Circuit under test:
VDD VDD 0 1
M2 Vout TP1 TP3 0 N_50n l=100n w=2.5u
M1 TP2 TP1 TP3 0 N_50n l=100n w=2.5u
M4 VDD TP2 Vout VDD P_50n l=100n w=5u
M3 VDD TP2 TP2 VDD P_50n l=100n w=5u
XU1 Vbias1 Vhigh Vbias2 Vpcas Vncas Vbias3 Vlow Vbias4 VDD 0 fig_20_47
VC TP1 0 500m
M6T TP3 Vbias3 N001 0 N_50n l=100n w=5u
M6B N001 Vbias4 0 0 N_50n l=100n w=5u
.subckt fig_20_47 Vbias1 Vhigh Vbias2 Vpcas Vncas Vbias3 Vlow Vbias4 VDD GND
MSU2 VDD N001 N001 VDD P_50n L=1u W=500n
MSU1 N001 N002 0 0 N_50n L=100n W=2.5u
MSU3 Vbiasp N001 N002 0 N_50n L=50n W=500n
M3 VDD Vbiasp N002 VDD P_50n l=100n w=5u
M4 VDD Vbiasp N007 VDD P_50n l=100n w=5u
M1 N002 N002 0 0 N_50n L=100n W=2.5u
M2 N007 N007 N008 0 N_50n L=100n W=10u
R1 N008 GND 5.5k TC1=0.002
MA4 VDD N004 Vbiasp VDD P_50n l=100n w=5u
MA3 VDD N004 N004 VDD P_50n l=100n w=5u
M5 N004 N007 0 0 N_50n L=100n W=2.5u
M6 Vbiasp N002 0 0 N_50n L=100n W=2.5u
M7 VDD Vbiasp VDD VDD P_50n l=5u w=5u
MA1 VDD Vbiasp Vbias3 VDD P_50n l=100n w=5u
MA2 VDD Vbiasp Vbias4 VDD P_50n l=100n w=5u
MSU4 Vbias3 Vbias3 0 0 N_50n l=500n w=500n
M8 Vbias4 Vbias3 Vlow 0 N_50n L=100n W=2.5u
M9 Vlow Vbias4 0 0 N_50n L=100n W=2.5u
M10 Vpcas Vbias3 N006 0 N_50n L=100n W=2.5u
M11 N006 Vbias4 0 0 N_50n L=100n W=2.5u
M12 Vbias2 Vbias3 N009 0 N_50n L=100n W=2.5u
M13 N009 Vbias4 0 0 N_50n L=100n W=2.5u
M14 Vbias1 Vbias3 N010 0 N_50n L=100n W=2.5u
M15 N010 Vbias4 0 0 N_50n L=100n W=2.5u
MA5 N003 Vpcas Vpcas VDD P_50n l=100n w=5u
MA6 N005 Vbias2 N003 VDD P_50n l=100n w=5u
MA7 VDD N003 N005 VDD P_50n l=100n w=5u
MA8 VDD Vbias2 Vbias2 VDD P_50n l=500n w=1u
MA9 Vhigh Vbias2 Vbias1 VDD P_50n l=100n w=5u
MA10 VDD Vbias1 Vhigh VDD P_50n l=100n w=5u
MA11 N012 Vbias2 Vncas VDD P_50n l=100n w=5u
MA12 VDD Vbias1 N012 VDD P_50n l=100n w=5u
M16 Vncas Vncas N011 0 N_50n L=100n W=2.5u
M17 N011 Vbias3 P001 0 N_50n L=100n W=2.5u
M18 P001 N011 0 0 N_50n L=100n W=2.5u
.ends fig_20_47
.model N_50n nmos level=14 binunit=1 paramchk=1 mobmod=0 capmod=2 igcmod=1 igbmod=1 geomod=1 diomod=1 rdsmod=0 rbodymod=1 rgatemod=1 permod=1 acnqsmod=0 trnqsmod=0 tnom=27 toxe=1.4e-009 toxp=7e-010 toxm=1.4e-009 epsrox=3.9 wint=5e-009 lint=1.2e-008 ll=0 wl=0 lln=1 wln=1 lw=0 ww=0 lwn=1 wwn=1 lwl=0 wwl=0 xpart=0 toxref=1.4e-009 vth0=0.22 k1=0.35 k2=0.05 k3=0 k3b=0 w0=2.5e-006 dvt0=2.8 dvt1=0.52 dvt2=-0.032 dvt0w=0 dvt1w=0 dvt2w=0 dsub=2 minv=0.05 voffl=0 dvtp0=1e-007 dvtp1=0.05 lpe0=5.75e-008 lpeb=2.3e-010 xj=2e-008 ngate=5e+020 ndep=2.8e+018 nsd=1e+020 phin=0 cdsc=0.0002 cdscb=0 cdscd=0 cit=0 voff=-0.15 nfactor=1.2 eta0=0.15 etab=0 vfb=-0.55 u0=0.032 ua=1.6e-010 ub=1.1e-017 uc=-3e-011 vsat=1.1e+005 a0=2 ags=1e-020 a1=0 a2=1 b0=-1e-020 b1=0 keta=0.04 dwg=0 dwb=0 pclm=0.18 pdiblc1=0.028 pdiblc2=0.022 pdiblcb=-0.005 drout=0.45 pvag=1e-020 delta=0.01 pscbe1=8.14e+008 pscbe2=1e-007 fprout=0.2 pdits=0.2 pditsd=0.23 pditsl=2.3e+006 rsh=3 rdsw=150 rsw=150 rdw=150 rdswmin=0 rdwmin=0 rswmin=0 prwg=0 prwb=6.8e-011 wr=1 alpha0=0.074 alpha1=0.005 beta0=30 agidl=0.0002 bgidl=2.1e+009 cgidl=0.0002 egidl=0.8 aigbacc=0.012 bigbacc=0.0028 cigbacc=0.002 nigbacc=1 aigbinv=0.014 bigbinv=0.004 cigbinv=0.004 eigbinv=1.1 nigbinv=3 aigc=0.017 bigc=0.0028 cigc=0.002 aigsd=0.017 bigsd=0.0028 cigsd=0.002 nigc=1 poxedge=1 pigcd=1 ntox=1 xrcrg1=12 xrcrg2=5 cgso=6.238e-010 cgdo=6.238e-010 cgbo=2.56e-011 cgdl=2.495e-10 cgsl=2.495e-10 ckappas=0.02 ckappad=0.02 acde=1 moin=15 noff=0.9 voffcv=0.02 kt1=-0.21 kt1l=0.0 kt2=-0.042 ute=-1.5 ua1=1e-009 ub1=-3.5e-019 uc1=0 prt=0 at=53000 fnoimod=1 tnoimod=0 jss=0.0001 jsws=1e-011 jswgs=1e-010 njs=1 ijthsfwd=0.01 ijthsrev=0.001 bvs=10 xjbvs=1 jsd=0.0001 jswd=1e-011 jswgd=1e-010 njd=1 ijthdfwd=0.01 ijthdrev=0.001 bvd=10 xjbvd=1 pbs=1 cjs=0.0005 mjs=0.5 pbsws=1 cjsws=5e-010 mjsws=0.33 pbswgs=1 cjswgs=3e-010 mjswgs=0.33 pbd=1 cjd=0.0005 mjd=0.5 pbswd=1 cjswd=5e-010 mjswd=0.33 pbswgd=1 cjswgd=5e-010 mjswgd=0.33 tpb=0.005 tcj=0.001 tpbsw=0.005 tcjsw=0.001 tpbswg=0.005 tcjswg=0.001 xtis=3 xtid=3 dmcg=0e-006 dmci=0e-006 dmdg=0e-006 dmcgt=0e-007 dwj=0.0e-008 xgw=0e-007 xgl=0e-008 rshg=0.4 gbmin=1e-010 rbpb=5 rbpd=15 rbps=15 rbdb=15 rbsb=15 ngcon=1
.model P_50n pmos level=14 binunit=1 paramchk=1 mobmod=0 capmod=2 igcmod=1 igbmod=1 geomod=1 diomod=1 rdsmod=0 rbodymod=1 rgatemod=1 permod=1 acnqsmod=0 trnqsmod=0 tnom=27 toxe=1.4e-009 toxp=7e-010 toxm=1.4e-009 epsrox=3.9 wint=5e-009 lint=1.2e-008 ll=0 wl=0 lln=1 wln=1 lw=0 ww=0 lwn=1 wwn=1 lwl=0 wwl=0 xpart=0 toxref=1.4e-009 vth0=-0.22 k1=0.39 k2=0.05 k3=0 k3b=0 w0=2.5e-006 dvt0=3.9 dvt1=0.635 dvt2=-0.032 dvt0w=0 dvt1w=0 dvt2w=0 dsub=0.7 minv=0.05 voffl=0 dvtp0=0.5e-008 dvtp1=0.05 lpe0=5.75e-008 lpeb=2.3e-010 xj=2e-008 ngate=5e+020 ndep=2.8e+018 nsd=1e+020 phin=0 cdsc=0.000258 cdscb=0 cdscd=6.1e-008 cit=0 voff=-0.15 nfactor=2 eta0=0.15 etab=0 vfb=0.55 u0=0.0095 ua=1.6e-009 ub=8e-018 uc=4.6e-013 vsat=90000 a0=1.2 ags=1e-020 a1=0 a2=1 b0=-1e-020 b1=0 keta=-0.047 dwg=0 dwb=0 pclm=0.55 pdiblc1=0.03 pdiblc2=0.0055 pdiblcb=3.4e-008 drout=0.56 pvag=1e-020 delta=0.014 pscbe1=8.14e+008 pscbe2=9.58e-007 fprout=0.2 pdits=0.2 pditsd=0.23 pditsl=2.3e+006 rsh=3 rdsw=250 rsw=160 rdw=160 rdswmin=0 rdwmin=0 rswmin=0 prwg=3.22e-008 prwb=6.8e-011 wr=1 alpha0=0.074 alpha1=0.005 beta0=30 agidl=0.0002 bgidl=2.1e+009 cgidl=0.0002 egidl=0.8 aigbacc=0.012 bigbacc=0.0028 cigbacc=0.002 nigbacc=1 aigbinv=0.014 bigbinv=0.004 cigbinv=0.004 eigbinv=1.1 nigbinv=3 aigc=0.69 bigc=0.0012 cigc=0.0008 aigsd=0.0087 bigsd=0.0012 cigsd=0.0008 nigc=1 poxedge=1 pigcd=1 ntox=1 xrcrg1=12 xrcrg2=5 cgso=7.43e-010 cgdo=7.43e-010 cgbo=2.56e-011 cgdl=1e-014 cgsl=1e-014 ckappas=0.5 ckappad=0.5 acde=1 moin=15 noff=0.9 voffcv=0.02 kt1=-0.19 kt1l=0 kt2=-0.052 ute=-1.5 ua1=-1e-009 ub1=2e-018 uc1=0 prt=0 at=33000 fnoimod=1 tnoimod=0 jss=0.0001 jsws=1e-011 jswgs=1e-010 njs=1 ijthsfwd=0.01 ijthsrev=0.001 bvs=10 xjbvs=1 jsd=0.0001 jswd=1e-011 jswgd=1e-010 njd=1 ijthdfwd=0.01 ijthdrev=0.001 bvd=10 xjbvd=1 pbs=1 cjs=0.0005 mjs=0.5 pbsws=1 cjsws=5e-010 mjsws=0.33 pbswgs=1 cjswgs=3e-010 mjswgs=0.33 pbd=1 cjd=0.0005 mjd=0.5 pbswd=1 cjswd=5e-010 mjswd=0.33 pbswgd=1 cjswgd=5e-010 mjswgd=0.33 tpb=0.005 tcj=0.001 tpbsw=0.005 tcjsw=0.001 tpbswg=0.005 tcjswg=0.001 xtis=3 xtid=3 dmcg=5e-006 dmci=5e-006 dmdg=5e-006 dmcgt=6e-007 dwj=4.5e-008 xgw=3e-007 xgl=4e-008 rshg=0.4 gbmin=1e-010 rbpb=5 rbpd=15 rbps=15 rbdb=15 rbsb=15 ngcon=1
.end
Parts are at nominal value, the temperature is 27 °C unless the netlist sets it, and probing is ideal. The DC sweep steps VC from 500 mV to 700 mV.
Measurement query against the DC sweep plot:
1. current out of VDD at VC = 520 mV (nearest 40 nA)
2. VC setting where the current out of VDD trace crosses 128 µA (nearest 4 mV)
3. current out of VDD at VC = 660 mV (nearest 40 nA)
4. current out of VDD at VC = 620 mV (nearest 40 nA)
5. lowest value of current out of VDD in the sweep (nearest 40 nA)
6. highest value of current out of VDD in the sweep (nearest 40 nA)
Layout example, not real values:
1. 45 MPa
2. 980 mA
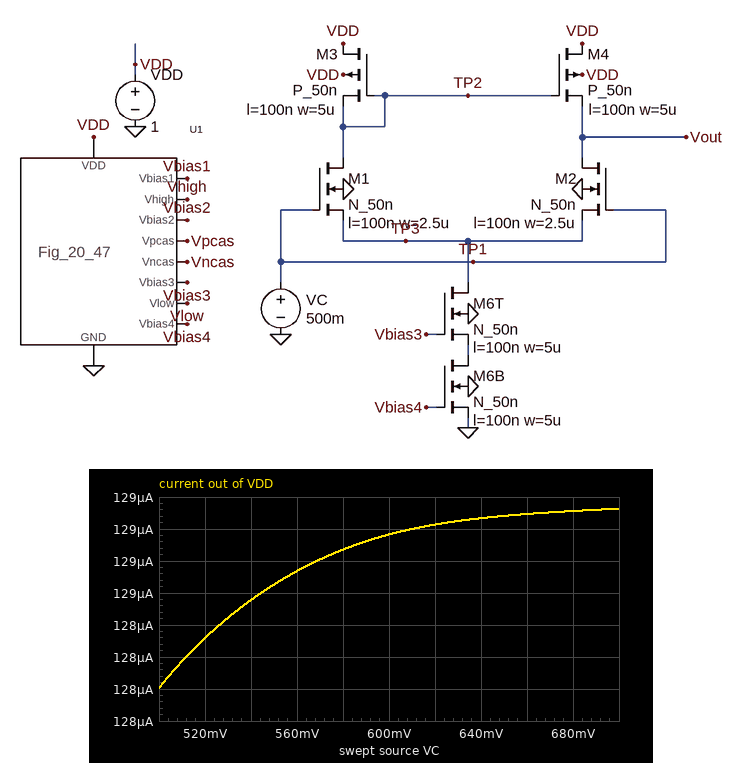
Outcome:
1. 128.32 µA
2. 512 mV
3. 129.08 µA
4. 129.04 µA
5. 128.00 µA
6. 129.12 µA
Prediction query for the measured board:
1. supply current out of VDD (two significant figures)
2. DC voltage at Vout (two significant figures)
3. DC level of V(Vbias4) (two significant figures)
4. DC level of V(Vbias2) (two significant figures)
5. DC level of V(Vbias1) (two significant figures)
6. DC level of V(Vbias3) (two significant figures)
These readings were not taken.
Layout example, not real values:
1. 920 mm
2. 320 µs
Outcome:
1. 130 µA
2. 650 mV
3. 360 mV
4. 370 mV
5. 640 mV
6. 540 mV
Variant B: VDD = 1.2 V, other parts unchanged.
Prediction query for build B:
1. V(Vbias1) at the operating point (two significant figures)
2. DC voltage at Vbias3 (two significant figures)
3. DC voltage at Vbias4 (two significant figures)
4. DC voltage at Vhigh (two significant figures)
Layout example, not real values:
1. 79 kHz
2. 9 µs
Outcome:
1. 840 mV
2. 550 mV
3. 360 mV
4. 980 mV
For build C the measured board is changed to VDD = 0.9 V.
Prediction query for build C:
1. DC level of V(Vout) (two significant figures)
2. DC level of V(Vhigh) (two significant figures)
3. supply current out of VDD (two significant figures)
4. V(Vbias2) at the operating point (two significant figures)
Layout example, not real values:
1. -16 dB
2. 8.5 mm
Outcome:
1. 550 mV
2. 690 mV
3. 120 µA
4. 270 mV
